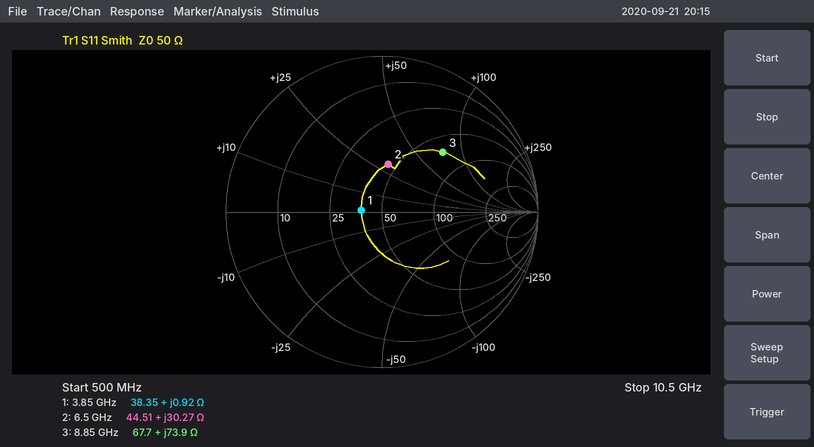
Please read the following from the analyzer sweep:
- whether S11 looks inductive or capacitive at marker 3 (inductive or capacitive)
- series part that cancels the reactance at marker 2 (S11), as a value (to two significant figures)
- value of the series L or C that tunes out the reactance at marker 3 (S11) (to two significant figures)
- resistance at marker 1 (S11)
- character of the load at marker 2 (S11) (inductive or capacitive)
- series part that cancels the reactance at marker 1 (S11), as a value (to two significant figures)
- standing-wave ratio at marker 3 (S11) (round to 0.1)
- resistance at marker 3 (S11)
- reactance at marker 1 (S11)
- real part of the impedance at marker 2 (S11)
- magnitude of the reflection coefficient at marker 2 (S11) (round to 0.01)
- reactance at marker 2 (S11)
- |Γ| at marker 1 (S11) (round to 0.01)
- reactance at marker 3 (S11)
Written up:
inductive
810 fF
240 fF
38.35 Ω
inductive
45 pF
3.4
67.7 Ω
+0.92 Ω
44.51 Ω
0.31
+30.27 Ω
0.13
+73.9 Ω
